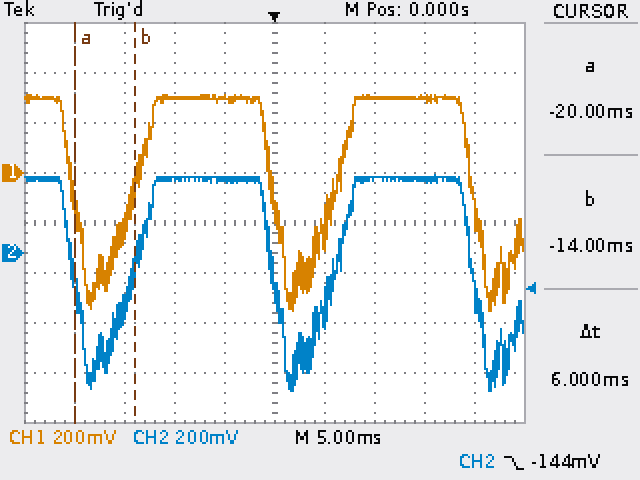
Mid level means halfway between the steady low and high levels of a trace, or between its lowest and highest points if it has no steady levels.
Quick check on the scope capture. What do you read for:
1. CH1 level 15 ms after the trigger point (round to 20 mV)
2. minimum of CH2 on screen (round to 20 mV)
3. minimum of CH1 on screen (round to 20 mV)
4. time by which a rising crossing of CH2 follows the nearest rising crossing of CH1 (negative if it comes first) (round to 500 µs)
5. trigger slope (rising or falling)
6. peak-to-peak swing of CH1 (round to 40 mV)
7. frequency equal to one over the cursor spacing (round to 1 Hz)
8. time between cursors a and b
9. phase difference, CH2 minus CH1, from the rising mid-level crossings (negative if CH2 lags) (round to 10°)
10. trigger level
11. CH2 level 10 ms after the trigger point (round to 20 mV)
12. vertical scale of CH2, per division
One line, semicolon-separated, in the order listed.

300 mV; -560 mV; -560 mV; 0.0 ms; falling; 880 mV; 167 Hz; 6 ms; 0°; -144 mV; 300 mV; 200 mV
